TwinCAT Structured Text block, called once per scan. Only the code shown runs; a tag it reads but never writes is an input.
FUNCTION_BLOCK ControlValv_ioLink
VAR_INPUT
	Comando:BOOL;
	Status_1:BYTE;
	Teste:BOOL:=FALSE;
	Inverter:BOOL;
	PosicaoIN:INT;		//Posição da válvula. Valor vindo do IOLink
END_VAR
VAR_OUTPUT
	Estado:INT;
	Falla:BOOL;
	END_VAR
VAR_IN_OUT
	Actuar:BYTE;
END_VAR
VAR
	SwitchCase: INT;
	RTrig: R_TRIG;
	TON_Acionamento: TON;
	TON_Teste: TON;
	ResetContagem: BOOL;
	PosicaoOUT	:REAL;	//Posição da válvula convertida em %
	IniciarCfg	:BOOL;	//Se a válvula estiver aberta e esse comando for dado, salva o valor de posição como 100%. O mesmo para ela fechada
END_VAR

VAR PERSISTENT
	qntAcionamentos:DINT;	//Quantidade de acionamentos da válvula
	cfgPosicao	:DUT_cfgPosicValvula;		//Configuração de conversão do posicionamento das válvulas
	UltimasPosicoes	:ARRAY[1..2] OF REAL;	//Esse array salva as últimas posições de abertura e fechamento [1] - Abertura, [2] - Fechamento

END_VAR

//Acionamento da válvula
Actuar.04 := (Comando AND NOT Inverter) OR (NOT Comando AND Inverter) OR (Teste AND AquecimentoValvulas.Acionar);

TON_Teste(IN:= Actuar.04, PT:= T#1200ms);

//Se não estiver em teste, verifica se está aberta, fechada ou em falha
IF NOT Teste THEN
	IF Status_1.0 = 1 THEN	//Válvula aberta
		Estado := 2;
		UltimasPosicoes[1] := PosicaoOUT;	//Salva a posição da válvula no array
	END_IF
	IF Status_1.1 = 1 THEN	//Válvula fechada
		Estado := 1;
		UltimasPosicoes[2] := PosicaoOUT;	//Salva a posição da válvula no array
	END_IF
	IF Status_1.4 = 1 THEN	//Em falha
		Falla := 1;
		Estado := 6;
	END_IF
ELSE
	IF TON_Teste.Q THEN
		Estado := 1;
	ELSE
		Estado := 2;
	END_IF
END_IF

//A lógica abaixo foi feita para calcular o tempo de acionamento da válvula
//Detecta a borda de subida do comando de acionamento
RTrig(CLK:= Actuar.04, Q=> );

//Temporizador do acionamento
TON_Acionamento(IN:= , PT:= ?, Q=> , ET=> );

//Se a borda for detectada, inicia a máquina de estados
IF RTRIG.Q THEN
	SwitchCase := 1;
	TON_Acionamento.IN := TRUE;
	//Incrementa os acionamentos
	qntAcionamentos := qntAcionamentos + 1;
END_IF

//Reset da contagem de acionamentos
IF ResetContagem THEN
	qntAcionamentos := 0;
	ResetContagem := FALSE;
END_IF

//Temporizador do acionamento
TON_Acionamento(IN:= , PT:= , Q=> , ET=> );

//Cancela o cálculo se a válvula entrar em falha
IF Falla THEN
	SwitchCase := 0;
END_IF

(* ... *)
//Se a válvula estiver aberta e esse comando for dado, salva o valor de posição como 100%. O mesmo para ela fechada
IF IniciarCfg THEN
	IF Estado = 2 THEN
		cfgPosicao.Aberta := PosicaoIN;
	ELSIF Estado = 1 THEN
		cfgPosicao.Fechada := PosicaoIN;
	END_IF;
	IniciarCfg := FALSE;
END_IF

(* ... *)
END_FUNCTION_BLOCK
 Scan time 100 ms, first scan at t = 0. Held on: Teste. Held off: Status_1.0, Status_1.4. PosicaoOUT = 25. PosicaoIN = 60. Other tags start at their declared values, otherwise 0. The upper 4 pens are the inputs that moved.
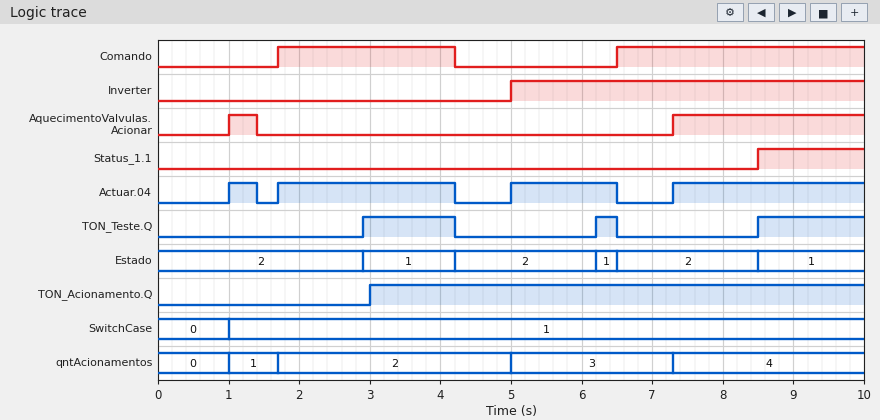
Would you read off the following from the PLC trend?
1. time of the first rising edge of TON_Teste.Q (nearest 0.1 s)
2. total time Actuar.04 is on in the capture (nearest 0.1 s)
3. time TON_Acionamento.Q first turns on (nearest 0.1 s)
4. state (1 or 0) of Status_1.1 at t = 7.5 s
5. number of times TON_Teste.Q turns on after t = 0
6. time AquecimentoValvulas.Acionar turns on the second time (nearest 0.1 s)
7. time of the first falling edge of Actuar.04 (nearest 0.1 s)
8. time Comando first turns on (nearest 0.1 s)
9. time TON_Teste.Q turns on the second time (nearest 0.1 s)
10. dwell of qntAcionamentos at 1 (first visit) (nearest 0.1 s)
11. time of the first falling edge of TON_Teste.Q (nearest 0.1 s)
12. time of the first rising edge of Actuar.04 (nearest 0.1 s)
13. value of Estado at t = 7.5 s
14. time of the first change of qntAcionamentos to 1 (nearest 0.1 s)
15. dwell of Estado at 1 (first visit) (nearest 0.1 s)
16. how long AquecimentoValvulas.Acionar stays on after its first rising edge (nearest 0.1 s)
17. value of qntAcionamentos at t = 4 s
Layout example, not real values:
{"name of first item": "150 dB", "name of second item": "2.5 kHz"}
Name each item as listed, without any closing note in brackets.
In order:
{"time of the first rising edge of TON_Teste.Q": "2.9 s", "total time Actuar.04 is on in the capture": "7.1 s", "time TON_Acionamento.Q first turns on": "3.0 s", "state (1 or 0) of Status_1.1 at t = 7.5 s": "0", "number of times TON_Teste.Q turns on after t = 0": "3", "time AquecimentoValvulas.Acionar turns on the second time": "7.3 s", "time of the first falling edge of Actuar.04": "1.4 s", "time Comando first turns on": "1.7 s", "time TON_Teste.Q turns on the second time": "6.2 s", "dwell of qntAcionamentos at 1 (first visit)": "0.7 s", "time of the first falling edge of TON_Teste.Q": "4.2 s", "time of the first rising edge of Actuar.04": "1.0 s", "value of Estado at t = 7.5 s": "2", "time of the first change of qntAcionamentos to 1": "1.0 s", "dwell of Estado at 1 (first visit)": "1.3 s", "how long AquecimentoValvulas.Acionar stays on after its first rising edge": "0.4 s", "value of qntAcionamentos at t = 4 s": "2"}
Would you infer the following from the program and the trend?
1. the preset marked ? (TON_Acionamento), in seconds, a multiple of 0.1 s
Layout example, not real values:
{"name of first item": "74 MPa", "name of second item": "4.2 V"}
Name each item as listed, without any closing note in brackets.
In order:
{"the preset marked ? (TON_Acionamento), in seconds, a multiple of 0.1 s": "2.0 s"}
